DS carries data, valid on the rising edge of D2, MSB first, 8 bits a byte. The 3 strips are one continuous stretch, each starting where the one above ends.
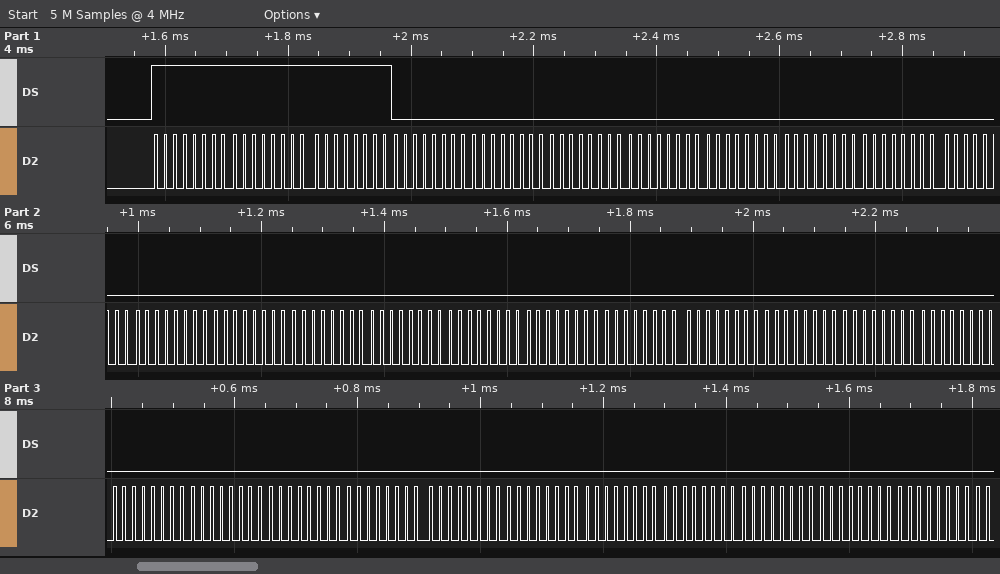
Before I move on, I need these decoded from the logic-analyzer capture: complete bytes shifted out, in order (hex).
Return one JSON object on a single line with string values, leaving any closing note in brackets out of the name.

{"complete bytes shifted out, in order": "FF FF FF 00 00 00 00 00 00 00 00 00 00 00 00 00 00 00 00 00 00 00 00 00 00 00 00 00 00 00 00 00 00"}
